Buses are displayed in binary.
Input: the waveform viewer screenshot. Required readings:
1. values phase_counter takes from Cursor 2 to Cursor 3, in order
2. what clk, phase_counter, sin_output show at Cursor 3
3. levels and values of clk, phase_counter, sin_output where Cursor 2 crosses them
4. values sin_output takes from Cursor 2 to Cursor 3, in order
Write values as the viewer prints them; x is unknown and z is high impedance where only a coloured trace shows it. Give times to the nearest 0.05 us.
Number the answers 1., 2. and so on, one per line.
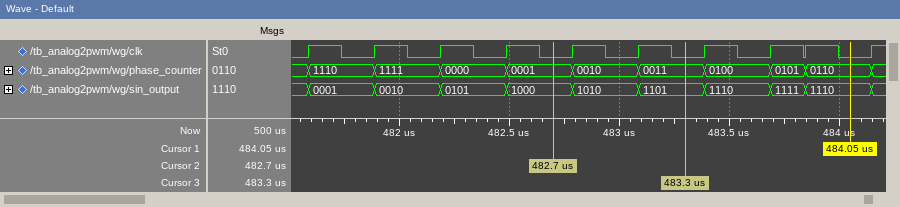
1. 0001, 0010, 0011
2. clk=0, phase_counter=0011, sin_output=1101
3. clk=0, phase_counter=0001, sin_output=1000
4. 1000, 1010, 1101
